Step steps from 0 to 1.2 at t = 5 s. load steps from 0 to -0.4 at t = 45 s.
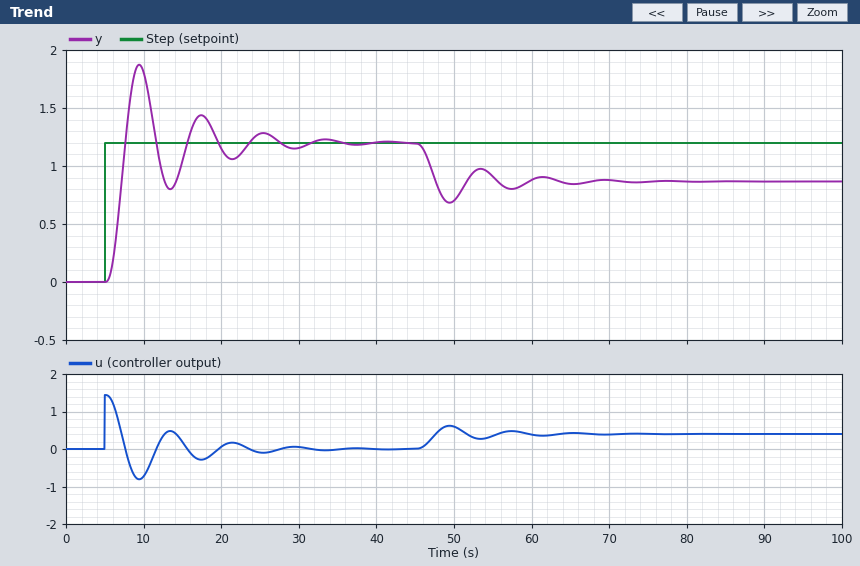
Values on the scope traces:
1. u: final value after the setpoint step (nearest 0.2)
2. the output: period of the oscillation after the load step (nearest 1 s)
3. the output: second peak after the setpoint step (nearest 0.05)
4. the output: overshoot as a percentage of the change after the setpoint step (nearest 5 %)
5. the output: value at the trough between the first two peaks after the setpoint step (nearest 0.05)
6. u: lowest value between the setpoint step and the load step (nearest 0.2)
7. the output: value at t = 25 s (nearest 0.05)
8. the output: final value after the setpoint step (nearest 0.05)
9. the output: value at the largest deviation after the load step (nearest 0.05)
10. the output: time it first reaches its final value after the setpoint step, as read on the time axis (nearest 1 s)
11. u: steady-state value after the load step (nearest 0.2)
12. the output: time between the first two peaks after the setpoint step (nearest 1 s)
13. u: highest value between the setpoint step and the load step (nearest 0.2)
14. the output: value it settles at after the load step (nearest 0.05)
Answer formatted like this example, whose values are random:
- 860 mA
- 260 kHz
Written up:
- 0.0
- 8 s
- 1.45
- 55 %
- 0.80
- -0.8
- 1.30
- 1.20
- 0.70
- 8 s
- 0.4
- 8 s
- 1.4
- 0.85
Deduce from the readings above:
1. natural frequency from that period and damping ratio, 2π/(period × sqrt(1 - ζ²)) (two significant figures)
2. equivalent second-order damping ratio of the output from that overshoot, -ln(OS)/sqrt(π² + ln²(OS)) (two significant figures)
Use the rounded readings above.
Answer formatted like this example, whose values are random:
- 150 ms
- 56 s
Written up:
- 0.80 rad/s
- 0.19
